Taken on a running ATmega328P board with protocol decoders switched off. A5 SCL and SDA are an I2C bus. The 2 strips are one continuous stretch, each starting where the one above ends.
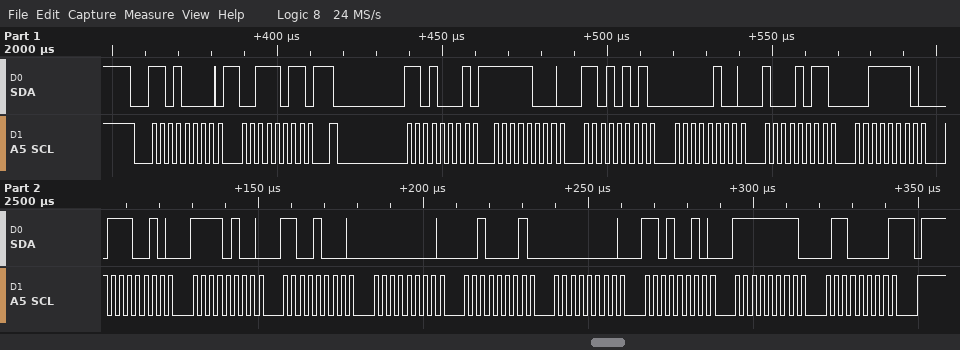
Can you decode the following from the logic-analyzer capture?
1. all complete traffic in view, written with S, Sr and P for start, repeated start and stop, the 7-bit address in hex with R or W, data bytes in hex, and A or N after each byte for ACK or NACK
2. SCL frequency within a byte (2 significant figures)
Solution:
S 68W A 3B A Sr 68R A F8 A D5 A 04 A 8B A 3E A 72 A F4 A C8 A 00 A 21 A 00 A D2 A FF A 60 N P
400 kHz
